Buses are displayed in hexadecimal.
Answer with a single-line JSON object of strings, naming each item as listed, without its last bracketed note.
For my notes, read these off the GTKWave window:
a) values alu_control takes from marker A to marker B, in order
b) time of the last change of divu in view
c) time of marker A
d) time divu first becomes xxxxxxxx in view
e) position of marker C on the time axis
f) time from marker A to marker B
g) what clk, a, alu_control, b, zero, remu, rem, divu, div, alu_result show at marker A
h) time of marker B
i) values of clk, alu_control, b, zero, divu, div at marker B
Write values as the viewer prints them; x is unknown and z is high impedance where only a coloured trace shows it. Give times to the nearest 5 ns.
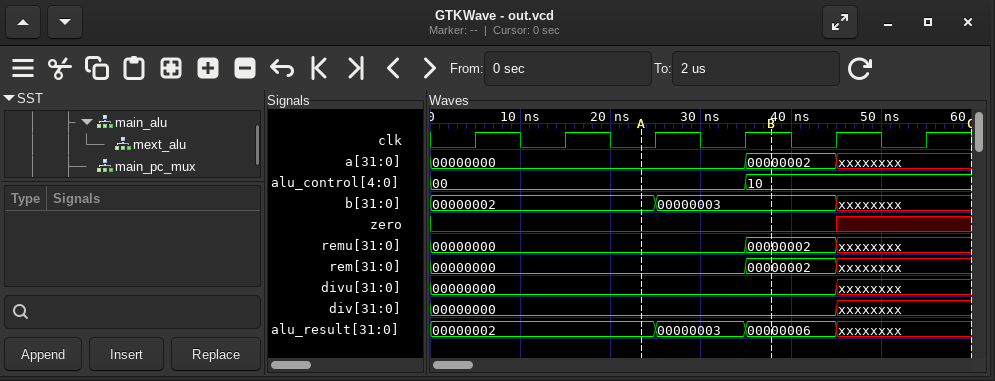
{"values alu_control takes from marker A to marker B, in order": "00, 10", "time of the last change of divu in view": "45 ns", "time of marker A": "25 ns", "time divu first becomes xxxxxxxx in view": "45 ns", "position of marker C on the time axis": "60 ns", "time from marker A to marker B": "15 ns", "what clk, a, alu_control, b, zero, remu, rem, divu, div, alu_result show at marker A": "clk=0, a=00000000, alu_control=00, b=00000002, zero=0, remu=00000000, rem=00000000, divu=00000000, div=00000000, alu_result=00000002", "time of marker B": "40 ns", "values of clk, alu_control, b, zero, divu, div at marker B": "clk=1, alu_control=10, b=00000003, zero=0, divu=00000000, div=00000000"}
